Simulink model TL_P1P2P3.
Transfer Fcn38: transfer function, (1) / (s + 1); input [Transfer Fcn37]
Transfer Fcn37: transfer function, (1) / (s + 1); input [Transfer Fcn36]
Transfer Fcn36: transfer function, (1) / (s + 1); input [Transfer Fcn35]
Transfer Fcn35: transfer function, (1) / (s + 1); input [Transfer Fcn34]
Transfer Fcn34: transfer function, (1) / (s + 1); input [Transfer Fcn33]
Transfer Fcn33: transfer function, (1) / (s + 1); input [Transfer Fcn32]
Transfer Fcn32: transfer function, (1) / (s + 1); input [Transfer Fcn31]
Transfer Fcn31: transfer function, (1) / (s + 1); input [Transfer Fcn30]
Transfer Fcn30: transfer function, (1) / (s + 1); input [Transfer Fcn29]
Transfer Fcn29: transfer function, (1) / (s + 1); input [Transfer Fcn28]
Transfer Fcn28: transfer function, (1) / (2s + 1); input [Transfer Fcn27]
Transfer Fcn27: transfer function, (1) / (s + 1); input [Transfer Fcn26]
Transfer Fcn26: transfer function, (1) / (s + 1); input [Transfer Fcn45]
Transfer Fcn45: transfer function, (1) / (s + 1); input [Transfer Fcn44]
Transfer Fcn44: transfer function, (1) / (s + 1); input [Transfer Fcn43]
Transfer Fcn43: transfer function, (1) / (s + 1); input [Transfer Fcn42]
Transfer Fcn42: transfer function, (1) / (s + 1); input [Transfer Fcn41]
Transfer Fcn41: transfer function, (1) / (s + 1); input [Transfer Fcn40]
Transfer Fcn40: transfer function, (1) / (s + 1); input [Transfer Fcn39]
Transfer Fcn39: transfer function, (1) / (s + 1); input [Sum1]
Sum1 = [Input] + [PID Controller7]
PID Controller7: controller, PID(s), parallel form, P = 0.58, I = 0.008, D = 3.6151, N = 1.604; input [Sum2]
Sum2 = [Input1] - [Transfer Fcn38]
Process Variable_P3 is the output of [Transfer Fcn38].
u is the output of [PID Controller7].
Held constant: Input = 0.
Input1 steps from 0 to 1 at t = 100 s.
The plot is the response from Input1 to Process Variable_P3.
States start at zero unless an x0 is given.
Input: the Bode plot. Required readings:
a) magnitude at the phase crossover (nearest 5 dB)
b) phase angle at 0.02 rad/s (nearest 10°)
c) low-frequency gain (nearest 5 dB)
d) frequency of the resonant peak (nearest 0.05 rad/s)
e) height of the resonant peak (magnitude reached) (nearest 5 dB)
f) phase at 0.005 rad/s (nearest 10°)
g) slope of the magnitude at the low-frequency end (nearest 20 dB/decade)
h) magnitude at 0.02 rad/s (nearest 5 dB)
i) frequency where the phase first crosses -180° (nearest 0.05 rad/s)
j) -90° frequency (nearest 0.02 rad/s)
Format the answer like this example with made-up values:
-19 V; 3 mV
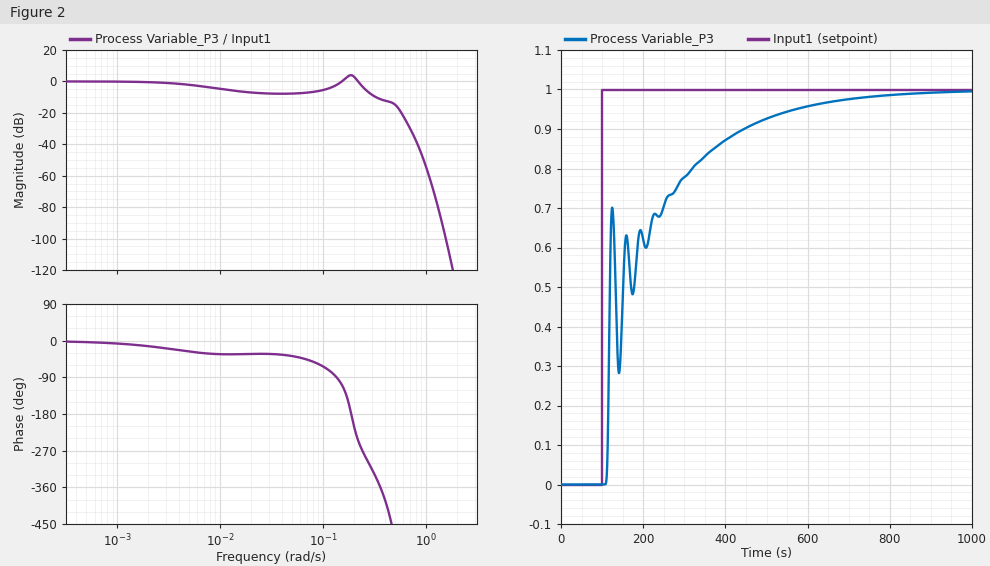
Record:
5 dB; -30°; 0 dB; 0.20 rad/s; 5 dB; -30°; 0 dB/decade; -5 dB; 0.20 rad/s; 0.14 rad/s
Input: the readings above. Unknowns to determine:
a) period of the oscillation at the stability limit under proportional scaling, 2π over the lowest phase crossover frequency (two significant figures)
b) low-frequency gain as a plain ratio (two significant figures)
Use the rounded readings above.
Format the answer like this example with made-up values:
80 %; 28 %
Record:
31 s; 1.0
